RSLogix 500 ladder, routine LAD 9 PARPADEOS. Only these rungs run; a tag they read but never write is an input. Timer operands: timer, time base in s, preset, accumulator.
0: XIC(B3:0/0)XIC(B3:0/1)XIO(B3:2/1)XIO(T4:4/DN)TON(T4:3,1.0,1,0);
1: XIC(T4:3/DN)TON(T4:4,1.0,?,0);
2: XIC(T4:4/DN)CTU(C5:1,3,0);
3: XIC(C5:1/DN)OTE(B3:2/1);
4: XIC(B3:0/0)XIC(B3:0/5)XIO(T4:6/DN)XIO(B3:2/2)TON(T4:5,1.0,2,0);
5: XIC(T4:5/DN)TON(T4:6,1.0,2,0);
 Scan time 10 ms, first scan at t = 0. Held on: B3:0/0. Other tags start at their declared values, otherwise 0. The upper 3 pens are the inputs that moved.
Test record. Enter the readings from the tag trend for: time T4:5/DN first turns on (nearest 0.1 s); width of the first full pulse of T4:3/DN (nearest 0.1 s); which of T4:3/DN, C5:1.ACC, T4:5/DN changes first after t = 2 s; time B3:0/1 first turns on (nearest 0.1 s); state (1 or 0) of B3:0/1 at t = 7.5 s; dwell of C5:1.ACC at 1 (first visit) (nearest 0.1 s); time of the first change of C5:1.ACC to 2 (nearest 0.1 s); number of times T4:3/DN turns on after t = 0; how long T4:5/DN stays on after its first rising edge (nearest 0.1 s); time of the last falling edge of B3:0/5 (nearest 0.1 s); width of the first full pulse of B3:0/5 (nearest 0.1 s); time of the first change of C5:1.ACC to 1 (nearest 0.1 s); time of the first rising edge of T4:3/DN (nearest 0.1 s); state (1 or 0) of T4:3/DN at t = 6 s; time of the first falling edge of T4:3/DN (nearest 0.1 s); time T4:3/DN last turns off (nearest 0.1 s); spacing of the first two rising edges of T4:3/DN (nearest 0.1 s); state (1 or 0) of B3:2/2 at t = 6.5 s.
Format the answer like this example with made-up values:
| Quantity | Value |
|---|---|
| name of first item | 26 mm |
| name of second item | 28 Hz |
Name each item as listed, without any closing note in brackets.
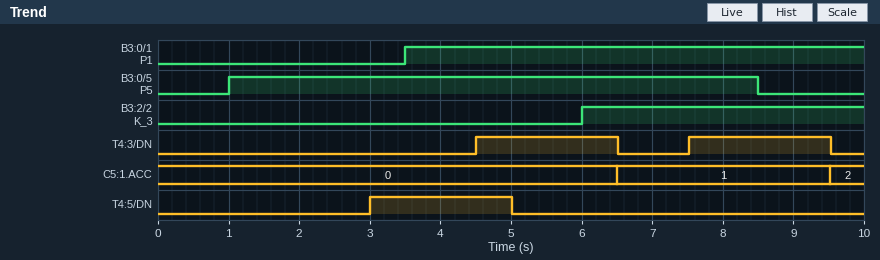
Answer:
| Quantity | Value |
|---|---|
| time T4:5/DN first turns on | 3.0 s |
| width of the first full pulse of T4:3/DN | 2.0 s |
| which of T4:3/DN, C5:1.ACC, T4:5/DN changes first after t = 2 s | T4:5/DN |
| time B3:0/1 first turns on | 3.5 s |
| state (1 or 0) of B3:0/1 at t = 7.5 s | 1 |
| dwell of C5:1.ACC at 1 (first visit) | 3.0 s |
| time of the first change of C5:1.ACC to 2 | 9.5 s |
| number of times T4:3/DN turns on after t = 0 | 2 |
| how long T4:5/DN stays on after its first rising edge | 2.0 s |
| time of the last falling edge of B3:0/5 | 8.5 s |
| width of the first full pulse of B3:0/5 | 7.5 s |
| time of the first change of C5:1.ACC to 1 | 6.5 s |
| time of the first rising edge of T4:3/DN | 4.5 s |
| state (1 or 0) of T4:3/DN at t = 6 s | 1 |
| time of the first falling edge of T4:3/DN | 6.5 s |
| time T4:3/DN last turns off | 9.5 s |
| spacing of the first two rising edges of T4:3/DN | 3.0 s |
| state (1 or 0) of B3:2/2 at t = 6.5 s | 1 |
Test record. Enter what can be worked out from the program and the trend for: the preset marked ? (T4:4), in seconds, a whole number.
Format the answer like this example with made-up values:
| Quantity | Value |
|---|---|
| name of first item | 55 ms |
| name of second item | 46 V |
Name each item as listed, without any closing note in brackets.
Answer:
| Quantity | Value |
|---|---|
| the preset marked ? (T4:4), in seconds, a whole number | 2 s |
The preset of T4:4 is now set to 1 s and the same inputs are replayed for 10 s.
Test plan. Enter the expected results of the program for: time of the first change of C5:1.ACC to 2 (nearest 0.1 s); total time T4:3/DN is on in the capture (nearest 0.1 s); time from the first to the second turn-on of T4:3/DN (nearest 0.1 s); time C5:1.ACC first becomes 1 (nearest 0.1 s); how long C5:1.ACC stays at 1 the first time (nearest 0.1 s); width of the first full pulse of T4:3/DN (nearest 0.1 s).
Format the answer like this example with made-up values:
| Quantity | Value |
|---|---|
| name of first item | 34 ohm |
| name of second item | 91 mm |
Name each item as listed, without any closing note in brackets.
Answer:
| Quantity | Value |
|---|---|
| time of the first change of C5:1.ACC to 2 | 7.5 s |
| total time T4:3/DN is on in the capture | 3.0 s |
| time from the first to the second turn-on of T4:3/DN | 2.0 s |
| time C5:1.ACC first becomes 1 | 5.5 s |
| how long C5:1.ACC stays at 1 the first time | 2.0 s |
| width of the first full pulse of T4:3/DN | 1.0 s |
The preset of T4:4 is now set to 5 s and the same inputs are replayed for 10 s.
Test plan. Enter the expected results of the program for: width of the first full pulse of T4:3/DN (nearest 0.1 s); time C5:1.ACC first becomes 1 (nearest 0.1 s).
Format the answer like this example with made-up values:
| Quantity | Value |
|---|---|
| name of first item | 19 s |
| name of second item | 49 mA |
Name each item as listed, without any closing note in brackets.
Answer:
| Quantity | Value |
|---|---|
| width of the first full pulse of T4:3/DN | 5.0 s |
| time C5:1.ACC first becomes 1 | 9.5 s |
